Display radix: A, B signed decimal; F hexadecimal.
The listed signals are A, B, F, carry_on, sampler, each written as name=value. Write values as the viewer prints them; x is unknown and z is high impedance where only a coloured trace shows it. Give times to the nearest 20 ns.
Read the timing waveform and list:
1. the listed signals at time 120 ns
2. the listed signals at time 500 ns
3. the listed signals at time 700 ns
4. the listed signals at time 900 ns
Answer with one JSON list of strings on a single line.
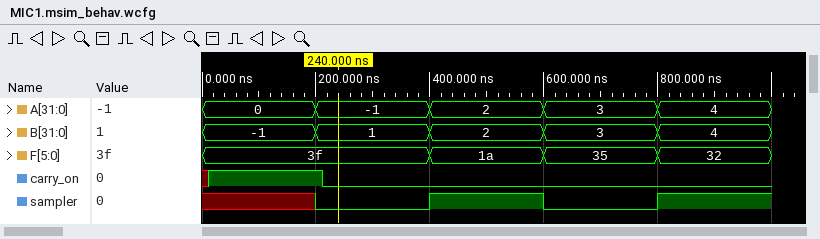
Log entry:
["A=0, B=-1, F=3f, carry_on=1, sampler=x", "A=2, B=2, F=1a, carry_on=0, sampler=1", "A=3, B=3, F=35, carry_on=0, sampler=0", "A=4, B=4, F=32, carry_on=0, sampler=1"]
